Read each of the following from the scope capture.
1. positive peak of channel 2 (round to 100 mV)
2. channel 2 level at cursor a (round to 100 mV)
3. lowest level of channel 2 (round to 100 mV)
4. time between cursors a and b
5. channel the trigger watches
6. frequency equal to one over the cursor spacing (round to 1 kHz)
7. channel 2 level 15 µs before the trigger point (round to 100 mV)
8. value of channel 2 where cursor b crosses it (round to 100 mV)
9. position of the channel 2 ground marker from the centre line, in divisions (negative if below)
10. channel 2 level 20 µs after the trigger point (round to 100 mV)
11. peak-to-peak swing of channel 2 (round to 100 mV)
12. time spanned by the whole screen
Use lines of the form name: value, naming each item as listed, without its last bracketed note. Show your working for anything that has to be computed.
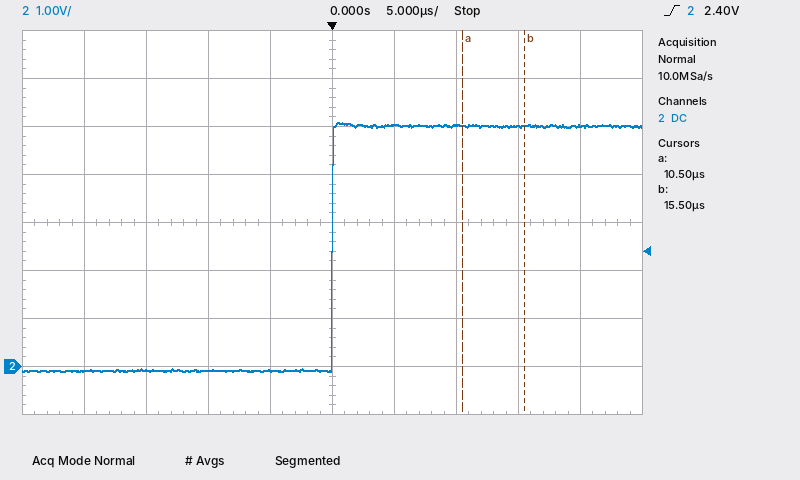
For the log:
positive peak of channel 2: 5.1 V
channel 2 level at cursor a: 5.0 V
lowest level of channel 2: -100 mV
time between cursors a and b: 15.5 µs − (10.5 µs) = 5.0 µs
channel the trigger watches: channel 2
frequency equal to one over the cursor spacing: 1 / 5.0 µs ≈ 200 kHz
channel 2 level 15 µs before the trigger point: -100 mV
value of channel 2 where cursor b crosses it: 5.0 V
position of the channel 2 ground marker from the centre line, in divisions: -3.0 div
channel 2 level 20 µs after the trigger point: 5.0 V
peak-to-peak swing of channel 2: 5.1 V − (-100 mV) = 5.2 V
time spanned by the whole screen: 50 µs
